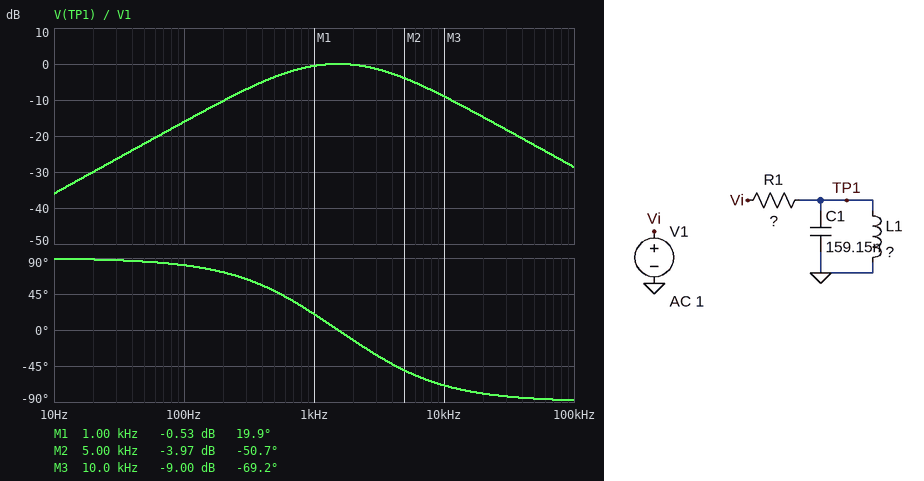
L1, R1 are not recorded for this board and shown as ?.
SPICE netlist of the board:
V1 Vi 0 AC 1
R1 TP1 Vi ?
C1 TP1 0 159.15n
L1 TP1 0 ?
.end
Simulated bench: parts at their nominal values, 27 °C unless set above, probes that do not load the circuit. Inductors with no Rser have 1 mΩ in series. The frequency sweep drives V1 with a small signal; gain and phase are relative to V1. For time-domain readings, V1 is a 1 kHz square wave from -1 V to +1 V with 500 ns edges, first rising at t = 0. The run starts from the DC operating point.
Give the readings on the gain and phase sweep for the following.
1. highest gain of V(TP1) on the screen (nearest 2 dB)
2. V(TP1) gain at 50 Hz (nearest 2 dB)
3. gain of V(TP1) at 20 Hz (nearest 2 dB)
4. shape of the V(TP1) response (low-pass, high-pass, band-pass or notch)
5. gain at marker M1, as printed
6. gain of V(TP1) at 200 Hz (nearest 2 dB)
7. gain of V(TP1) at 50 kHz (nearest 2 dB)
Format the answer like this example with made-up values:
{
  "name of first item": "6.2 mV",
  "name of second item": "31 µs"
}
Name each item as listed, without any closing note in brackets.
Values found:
{
  "highest gain of V(TP1) on the screen": "0 dB",
  "V(TP1) gain at 50 Hz": "-22 dB",
  "gain of V(TP1) at 20 Hz": "-30 dB",
  "shape of the V(TP1) response": "band-pass",
  "gain at marker M1, as printed": "-0.53 dB",
  "gain of V(TP1) at 200 Hz": "-10 dB",
  "gain of V(TP1) at 50 kHz": "-22 dB"
}
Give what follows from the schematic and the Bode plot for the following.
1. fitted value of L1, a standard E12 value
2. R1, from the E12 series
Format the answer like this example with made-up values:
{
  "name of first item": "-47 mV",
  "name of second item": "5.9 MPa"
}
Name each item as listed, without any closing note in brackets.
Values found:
{
  "fitted value of L1, a standard E12 value": "68 mH",
  "R1, from the E12 series": "270 Ω"
}
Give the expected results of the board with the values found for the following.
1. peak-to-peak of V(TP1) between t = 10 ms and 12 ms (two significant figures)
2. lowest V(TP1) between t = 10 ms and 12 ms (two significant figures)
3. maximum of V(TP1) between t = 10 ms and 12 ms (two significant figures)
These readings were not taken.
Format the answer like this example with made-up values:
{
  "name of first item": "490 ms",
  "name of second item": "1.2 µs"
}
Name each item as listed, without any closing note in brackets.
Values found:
{
  "peak-to-peak of V(TP1) between t = 10 ms and 12 ms": "2.8 V",
  "lowest V(TP1) between t = 10 ms and 12 ms": "-1.4 V",
  "maximum of V(TP1) between t = 10 ms and 12 ms": "1.4 V"
}
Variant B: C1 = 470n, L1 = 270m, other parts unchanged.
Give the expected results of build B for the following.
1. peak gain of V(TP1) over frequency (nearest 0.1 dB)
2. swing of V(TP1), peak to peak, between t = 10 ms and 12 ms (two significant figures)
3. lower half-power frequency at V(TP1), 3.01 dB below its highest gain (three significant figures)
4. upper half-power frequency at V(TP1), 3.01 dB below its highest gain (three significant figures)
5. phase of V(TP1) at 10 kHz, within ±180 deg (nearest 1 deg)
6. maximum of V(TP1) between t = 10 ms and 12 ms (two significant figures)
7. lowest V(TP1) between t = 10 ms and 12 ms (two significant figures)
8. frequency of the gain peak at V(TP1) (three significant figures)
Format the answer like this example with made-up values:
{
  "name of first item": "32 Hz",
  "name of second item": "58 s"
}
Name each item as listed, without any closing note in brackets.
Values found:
{
  "peak gain of V(TP1) over frequency": "0 dB",
  "swing of V(TP1), peak to peak, between t = 10 ms and 12 ms": "1.9 V",
  "lower half-power frequency at V(TP1), 3.01 dB below its highest gain": "143 Hz",
  "upper half-power frequency at V(TP1), 3.01 dB below its highest gain": "1.40 kHz",
  "phase of V(TP1) at 10 kHz, within ±180 deg": "-83 deg",
  "maximum of V(TP1) between t = 10 ms and 12 ms": "960 mV",
  "lowest V(TP1) between t = 10 ms and 12 ms": "-960 mV",
  "frequency of the gain peak at V(TP1)": "447 Hz"
}
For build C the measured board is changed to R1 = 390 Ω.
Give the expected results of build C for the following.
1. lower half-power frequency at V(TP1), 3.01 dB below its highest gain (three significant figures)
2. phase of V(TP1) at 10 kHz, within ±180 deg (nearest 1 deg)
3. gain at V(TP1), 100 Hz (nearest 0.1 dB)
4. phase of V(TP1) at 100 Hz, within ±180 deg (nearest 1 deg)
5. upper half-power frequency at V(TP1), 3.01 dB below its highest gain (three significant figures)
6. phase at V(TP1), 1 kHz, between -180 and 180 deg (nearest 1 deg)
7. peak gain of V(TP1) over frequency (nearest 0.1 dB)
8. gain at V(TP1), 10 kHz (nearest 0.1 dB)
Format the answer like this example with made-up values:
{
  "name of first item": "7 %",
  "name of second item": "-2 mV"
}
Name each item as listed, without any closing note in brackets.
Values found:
{
  "lower half-power frequency at V(TP1), 3.01 dB below its highest gain": "714 Hz",
  "phase of V(TP1) at 10 kHz, within ±180 deg": "-75 deg",
  "gain at V(TP1), 100 Hz": "-19.2 dB",
  "phase of V(TP1) at 100 Hz, within ±180 deg": "84 deg",
  "upper half-power frequency at V(TP1), 3.01 dB below its highest gain": "3.28 kHz",
  "phase at V(TP1), 1 kHz, between -180 and 180 deg": "28 deg",
  "peak gain of V(TP1) over frequency": "0 dB",
  "gain at V(TP1), 10 kHz": "-11.9 dB"
}
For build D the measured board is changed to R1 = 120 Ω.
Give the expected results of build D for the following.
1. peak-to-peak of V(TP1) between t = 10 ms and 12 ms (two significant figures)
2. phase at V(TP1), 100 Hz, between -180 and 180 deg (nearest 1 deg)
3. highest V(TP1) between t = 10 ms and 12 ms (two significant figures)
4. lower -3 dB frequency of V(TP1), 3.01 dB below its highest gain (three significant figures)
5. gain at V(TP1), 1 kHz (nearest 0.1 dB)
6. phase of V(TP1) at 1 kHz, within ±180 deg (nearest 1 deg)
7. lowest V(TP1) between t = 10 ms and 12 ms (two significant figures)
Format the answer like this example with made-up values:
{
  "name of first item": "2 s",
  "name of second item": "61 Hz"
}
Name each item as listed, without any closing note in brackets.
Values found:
{
  "peak-to-peak of V(TP1) between t = 10 ms and 12 ms": "2.6 V",
  "phase at V(TP1), 100 Hz, between -180 and 180 deg": "70 deg",
  "highest V(TP1) between t = 10 ms and 12 ms": "1.3 V",
  "lower -3 dB frequency of V(TP1), 3.01 dB below its highest gain": "272 Hz",
  "gain at V(TP1), 1 kHz": "-0.1 dB",
  "phase of V(TP1) at 1 kHz, within ±180 deg": "9 deg",
  "lowest V(TP1) between t = 10 ms and 12 ms": "-1.3 V"
}
